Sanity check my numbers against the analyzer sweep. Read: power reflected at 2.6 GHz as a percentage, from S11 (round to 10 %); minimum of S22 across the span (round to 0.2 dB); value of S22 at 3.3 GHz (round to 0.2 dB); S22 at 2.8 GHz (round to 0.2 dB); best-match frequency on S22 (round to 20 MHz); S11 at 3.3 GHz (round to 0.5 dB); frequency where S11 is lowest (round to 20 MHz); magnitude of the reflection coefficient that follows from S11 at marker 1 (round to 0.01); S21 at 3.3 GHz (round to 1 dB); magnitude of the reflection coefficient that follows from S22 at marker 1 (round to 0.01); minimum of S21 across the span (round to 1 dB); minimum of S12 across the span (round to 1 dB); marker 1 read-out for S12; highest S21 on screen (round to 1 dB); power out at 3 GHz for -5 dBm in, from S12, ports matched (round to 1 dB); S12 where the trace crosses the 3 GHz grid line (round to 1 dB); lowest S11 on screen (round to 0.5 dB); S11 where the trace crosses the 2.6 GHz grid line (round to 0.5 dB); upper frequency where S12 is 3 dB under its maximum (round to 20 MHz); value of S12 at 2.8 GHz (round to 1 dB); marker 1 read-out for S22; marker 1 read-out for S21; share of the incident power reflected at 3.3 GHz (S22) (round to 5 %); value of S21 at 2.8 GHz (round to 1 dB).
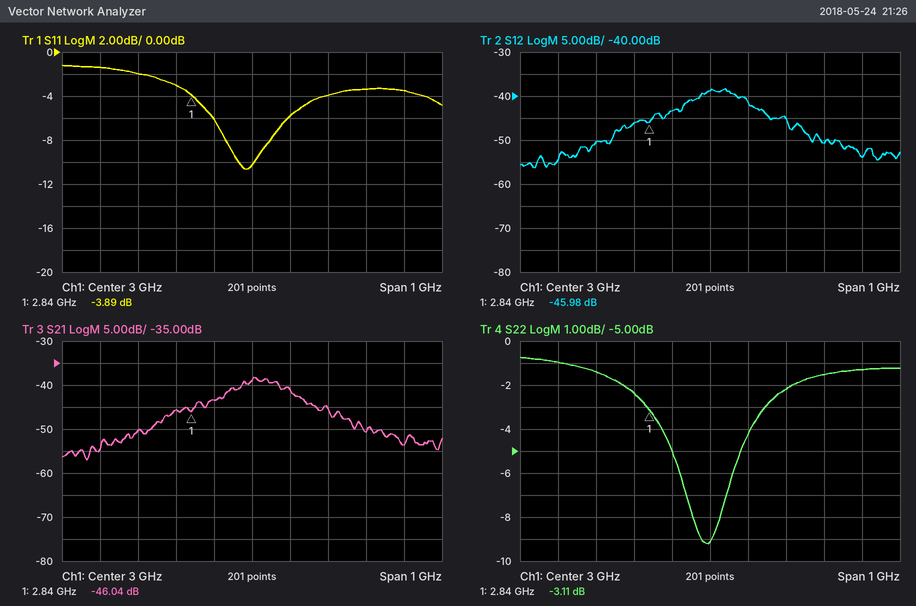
70 %
-9.2 dB
-1.6 dB
-2.4 dB
3.00 GHz
-3.5 dB
2.98 GHz
0.64
-51 dB
0.70
-57 dB
-56 dB
-45.98 dB
-38 dB
-44 dBm
-39 dB
-10.5 dB
-1.5 dB
3.10 GHz
-46 dB
-3.11 dB
-46.04 dB
70 %
-46 dB
